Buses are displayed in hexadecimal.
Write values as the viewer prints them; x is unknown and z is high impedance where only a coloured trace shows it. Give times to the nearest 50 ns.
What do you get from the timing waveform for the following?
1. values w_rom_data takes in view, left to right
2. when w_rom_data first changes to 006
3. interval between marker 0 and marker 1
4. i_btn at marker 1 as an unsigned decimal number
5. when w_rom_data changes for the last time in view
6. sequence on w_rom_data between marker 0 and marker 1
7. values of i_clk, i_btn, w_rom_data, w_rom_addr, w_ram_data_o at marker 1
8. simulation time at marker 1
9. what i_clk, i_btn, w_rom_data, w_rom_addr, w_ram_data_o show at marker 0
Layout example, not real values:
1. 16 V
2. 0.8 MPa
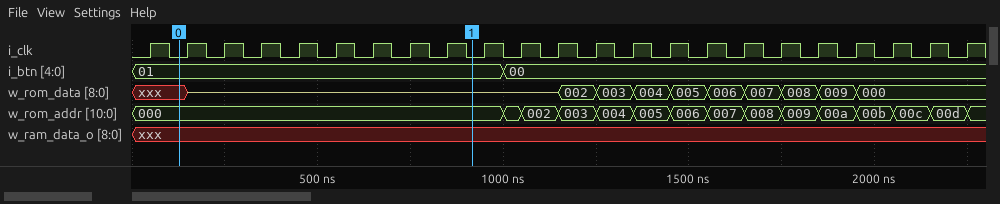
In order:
1. xxx, z, 002, 003, 004, 005, 006, 007, 008, 009, 000
2. 1550 ns
3. 800 ns
4. 1
5. 1950 ns
6. xxx, z
7. i_clk=0, i_btn=01, w_rom_data=z, w_rom_addr=000, w_ram_data_o=xxx
8. 900 ns
9. i_clk=0, i_btn=01, w_rom_data=xxx, w_rom_addr=000, w_ram_data_o=xxx
